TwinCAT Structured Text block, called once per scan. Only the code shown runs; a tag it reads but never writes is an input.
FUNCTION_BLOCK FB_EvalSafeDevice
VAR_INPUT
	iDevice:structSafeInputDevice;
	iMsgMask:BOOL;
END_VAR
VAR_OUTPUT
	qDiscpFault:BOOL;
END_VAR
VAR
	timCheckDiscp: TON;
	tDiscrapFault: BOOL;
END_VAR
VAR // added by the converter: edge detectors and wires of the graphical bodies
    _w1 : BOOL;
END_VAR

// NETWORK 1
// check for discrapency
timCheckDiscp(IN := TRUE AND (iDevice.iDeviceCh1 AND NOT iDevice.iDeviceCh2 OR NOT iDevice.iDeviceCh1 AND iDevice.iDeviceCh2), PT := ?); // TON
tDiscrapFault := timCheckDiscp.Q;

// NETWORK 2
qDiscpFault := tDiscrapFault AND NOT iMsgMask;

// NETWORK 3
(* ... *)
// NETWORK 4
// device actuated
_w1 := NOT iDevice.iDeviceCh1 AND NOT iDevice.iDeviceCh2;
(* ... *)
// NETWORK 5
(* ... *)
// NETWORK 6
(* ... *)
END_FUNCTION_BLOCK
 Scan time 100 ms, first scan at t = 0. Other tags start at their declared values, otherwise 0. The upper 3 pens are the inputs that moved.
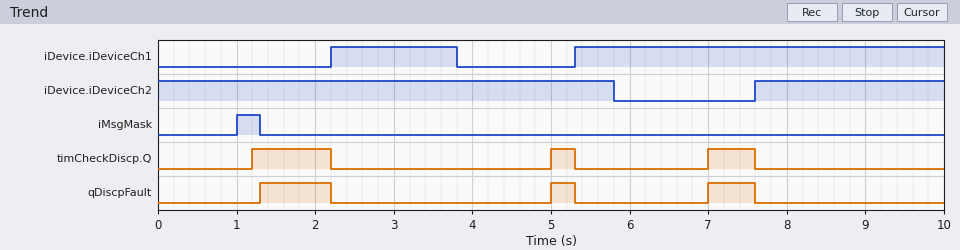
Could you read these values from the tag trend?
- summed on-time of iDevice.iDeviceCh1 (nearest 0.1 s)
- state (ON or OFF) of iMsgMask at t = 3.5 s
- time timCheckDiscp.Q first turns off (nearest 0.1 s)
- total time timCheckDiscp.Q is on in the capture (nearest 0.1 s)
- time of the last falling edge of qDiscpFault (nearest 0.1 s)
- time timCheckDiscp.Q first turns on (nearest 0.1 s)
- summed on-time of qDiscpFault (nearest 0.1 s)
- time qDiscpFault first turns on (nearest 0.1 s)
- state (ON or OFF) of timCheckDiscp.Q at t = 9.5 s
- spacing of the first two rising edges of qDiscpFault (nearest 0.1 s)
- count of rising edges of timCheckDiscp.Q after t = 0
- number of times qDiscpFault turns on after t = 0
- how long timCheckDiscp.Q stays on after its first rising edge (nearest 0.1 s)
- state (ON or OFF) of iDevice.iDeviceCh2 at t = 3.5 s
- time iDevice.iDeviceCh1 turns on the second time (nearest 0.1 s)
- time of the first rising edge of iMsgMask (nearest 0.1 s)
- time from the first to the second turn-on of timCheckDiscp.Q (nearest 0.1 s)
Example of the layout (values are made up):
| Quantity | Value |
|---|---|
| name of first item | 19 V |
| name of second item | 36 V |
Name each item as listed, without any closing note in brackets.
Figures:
| Quantity | Value |
|---|---|
| summed on-time of iDevice.iDeviceCh1 | 6.3 s |
| state (ON or OFF) of iMsgMask at t = 3.5 s | OFF |
| time timCheckDiscp.Q first turns off | 2.2 s |
| total time timCheckDiscp.Q is on in the capture | 1.9 s |
| time of the last falling edge of qDiscpFault | 7.6 s |
| time timCheckDiscp.Q first turns on | 1.2 s |
| summed on-time of qDiscpFault | 1.8 s |
| time qDiscpFault first turns on | 1.3 s |
| state (ON or OFF) of timCheckDiscp.Q at t = 9.5 s | OFF |
| spacing of the first two rising edges of qDiscpFault | 3.7 s |
| count of rising edges of timCheckDiscp.Q after t = 0 | 3 |
| number of times qDiscpFault turns on after t = 0 | 3 |
| how long timCheckDiscp.Q stays on after its first rising edge | 1.0 s |
| state (ON or OFF) of iDevice.iDeviceCh2 at t = 3.5 s | ON |
| time iDevice.iDeviceCh1 turns on the second time | 5.3 s |
| time of the first rising edge of iMsgMask | 1.0 s |
| time from the first to the second turn-on of timCheckDiscp.Q | 3.8 s |
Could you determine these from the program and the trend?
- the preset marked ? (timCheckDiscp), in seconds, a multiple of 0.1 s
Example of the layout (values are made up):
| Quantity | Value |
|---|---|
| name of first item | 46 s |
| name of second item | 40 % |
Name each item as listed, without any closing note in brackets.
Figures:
| Quantity | Value |
|---|---|
| the preset marked ? (timCheckDiscp), in seconds, a multiple of 0.1 s | 1.2 s |
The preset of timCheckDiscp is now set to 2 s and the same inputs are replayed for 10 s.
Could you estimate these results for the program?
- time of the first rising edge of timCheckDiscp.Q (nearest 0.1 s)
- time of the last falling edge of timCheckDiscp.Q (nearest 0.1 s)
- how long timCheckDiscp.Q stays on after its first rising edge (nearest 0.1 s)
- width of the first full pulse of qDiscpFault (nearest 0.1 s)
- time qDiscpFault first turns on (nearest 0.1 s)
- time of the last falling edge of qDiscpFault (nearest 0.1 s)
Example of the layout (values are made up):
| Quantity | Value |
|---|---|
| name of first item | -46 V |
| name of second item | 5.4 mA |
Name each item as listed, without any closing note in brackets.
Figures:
| Quantity | Value |
|---|---|
| time of the first rising edge of timCheckDiscp.Q | 2.0 s |
| time of the last falling edge of timCheckDiscp.Q | 2.2 s |
| how long timCheckDiscp.Q stays on after its first rising edge | 0.2 s |
| width of the first full pulse of qDiscpFault | 0.2 s |
| time qDiscpFault first turns on | 2.0 s |
| time of the last falling edge of qDiscpFault | 2.2 s |
